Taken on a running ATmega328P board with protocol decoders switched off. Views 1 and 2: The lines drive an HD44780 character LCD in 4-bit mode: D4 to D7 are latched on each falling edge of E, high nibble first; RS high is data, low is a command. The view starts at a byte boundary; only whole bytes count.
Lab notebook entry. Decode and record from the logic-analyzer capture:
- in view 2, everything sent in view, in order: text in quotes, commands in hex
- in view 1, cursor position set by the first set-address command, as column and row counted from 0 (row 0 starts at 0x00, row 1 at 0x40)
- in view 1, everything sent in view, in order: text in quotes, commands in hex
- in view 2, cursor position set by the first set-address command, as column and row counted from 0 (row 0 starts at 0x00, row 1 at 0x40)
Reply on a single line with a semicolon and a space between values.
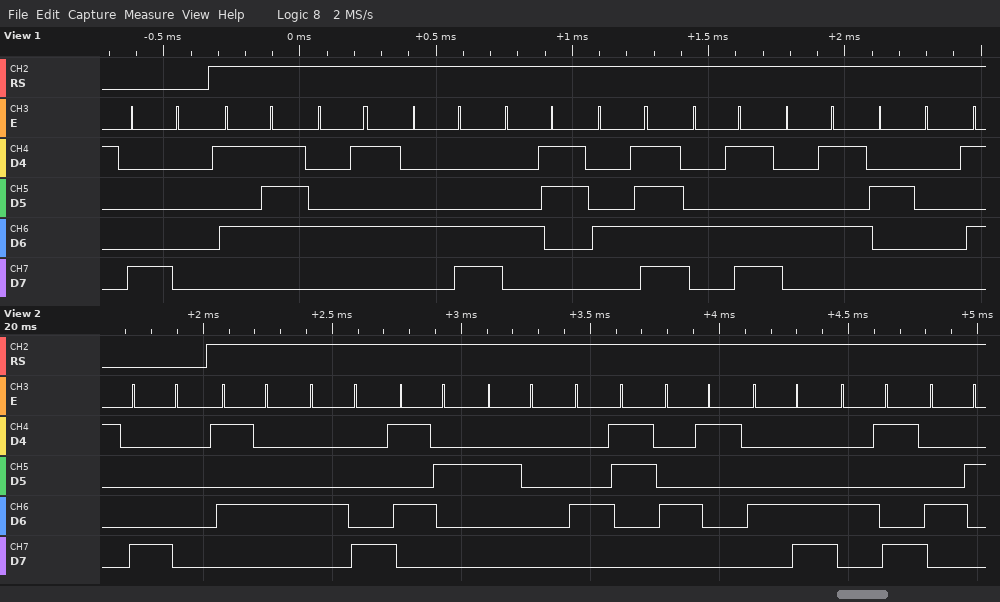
0x80 "THR CALIB"; column 0, row 0; 0x80 "WELCOME "; column 0, row 0
